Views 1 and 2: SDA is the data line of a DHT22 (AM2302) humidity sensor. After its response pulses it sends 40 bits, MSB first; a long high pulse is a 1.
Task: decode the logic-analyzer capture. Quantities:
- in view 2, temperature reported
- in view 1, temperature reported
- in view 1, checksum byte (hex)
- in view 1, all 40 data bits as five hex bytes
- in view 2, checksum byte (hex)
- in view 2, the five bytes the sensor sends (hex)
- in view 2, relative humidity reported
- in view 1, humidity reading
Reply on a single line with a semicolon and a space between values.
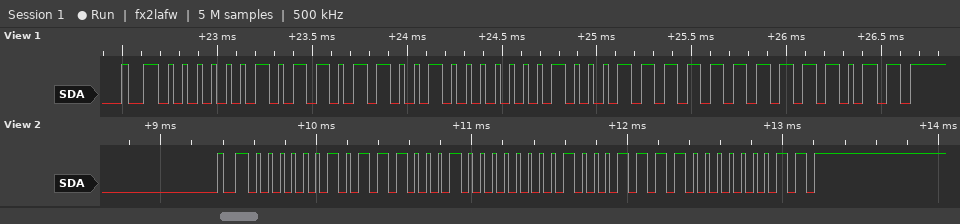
28.6 °C; 28.7 °C; 0xFB; 02 D9 01 1F FB; 0x03; 02 E2 01 1E 03; 73.8 %; 72.9 %
